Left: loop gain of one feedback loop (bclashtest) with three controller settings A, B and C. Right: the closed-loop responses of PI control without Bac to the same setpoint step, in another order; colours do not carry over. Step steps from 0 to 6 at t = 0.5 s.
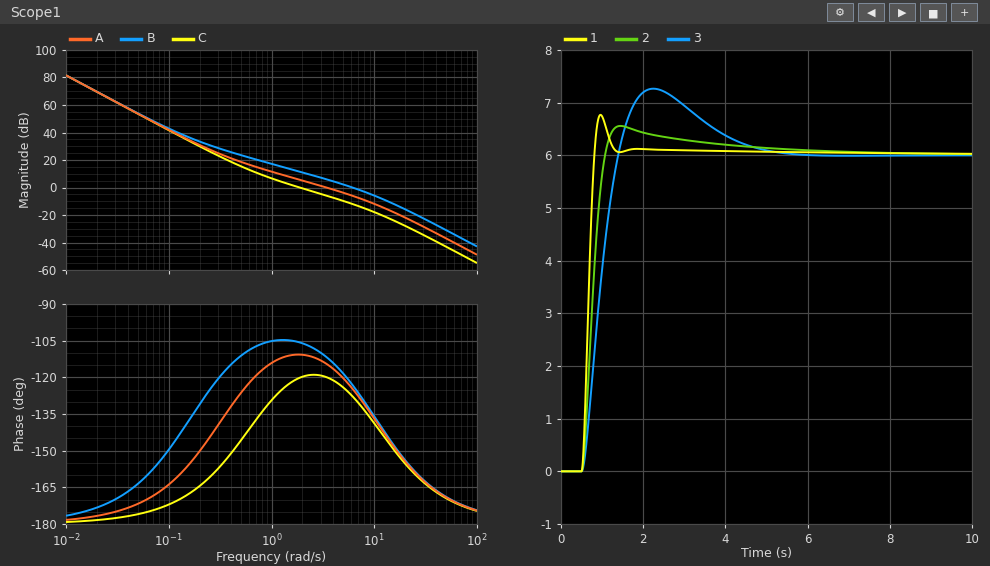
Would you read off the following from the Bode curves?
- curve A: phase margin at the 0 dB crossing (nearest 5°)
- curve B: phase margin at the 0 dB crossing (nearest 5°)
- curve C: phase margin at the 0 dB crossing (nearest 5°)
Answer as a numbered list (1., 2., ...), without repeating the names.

1. 65°
2. 55°
3. 60°
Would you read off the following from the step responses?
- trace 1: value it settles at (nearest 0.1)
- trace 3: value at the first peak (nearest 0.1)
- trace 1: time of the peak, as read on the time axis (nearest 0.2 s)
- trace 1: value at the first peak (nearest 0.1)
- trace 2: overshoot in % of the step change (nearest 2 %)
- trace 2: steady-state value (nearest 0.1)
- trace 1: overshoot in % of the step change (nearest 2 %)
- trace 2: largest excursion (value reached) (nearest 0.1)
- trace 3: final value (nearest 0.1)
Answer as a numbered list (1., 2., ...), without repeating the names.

1. 6.0
2. 7.3
3. 1.0 s
4. 6.8
5. 10 %
6. 6.0
7. 12 %
8. 6.6
9. 6.0
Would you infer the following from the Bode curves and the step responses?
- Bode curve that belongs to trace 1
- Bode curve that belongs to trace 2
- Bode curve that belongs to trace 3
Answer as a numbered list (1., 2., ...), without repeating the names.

1. B
2. A
3. C
